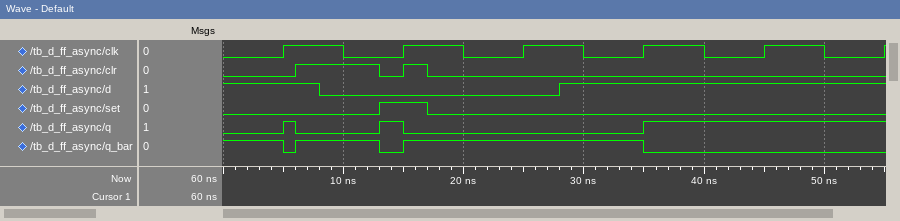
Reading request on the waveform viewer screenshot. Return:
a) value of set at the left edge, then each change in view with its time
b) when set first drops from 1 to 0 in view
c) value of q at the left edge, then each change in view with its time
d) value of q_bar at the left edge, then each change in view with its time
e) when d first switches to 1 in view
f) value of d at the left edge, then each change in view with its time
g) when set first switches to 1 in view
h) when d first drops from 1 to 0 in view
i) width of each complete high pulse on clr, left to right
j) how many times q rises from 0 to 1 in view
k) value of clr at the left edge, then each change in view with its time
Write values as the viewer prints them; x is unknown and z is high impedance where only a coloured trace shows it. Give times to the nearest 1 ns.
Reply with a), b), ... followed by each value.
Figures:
a) 0, 1 at 13 ns, 0 at 17 ns
b) 17 ns
c) 0, 1 at 5 ns, 0 at 6 ns, 1 at 13 ns, 0 at 15 ns, 1 at 35 ns
d) 1, 0 at 5 ns, 1 at 6 ns, 0 at 13 ns, 1 at 15 ns, 0 at 35 ns
e) 28 ns
f) 1, 0 at 8 ns, 1 at 28 ns
g) 13 ns
h) 8 ns
i) 7 ns, 2 ns
j) 3
k) 0, 1 at 6 ns, 0 at 13 ns, 1 at 15 ns, 0 at 17 ns
